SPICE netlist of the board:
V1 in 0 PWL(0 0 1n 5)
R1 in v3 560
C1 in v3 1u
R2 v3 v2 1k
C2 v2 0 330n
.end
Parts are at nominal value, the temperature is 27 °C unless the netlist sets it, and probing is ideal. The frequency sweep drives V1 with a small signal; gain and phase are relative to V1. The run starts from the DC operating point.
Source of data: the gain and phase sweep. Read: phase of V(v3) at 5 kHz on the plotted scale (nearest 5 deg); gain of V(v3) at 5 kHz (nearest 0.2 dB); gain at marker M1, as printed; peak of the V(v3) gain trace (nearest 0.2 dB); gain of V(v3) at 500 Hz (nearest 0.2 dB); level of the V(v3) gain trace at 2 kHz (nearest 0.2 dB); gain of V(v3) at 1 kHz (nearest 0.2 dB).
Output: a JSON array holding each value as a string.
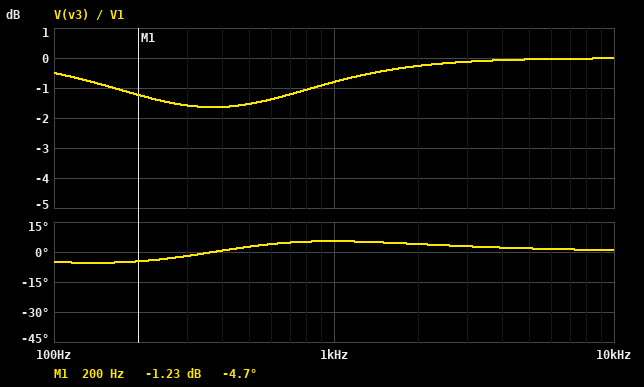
["0 deg", "0 dB", "-1.23 dB", "0 dB", "-1.6 dB", "-0.2 dB", "-0.8 dB"]
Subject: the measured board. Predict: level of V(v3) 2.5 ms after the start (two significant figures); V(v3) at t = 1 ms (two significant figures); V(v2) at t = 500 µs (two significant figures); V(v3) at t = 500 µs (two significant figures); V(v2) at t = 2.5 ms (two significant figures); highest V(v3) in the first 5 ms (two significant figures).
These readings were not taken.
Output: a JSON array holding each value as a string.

["4.9 V", "4.6 V", "3.4 V", "4.3 V", "4.9 V", "5.0 V"]
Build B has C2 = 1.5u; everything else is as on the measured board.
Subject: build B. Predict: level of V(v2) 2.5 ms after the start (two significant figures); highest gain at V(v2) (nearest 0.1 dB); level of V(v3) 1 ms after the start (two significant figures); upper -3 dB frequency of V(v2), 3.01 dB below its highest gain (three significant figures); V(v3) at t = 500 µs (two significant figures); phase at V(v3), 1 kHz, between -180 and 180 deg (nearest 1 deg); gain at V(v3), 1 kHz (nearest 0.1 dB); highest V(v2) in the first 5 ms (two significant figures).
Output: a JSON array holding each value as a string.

["3.3 V", "0 dB", "3.8 V", "63.8 Hz", "3.9 V", "8 deg", "-0.6 dB", "4.4 V"]
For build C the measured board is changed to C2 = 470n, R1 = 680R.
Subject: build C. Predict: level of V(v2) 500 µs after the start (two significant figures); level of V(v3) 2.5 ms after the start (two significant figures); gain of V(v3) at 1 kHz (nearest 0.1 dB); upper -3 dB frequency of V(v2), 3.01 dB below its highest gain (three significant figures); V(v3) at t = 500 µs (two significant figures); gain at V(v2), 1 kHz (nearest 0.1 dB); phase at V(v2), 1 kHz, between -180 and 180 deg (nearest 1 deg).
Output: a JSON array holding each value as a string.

["2.8 V", "4.8 V", "-0.7 dB", "186 Hz", "4.1 V", "-10.6 dB", "-65 deg"]
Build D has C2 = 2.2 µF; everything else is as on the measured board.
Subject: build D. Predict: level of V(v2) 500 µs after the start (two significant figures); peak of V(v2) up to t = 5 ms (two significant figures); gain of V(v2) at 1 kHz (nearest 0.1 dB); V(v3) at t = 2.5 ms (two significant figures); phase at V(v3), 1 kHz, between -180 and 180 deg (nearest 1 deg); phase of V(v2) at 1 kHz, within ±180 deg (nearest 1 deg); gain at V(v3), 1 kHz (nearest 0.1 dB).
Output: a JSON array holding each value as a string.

["860 mV", "3.8 V", "-23.4 dB", "4.1 V", "8 deg", "-78 deg", "-0.5 dB"]
